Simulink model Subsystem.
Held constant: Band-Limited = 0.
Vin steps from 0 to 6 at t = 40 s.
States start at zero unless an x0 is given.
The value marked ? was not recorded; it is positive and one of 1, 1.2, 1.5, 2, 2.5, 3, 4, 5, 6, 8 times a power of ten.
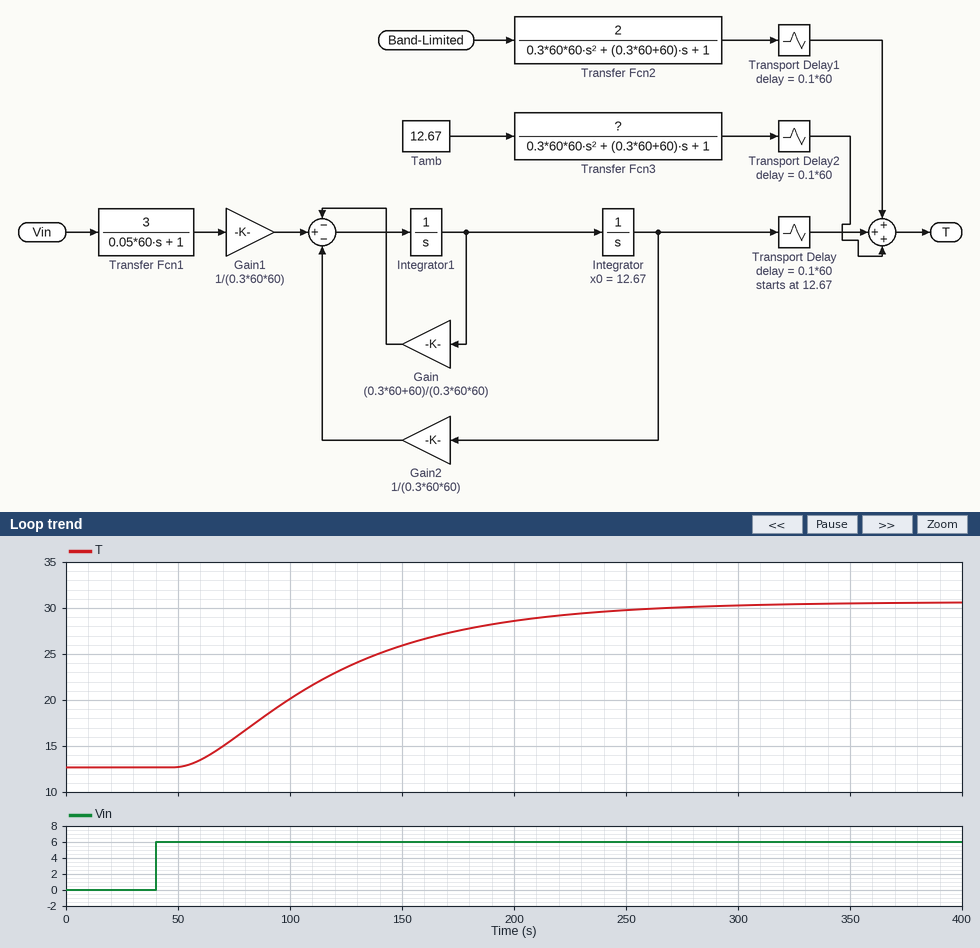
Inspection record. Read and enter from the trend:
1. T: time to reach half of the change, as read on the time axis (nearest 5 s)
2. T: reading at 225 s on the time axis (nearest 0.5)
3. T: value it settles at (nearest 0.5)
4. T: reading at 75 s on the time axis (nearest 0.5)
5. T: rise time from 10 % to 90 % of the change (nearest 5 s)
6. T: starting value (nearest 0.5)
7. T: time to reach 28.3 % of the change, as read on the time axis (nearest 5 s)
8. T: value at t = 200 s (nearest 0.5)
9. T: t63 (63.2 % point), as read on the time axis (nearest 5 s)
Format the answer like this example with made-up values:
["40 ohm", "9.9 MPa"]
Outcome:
["110 s", "29.5", "30.5", "16.0", "140 s", "12.5", "85 s", "28.5", "130 s"]
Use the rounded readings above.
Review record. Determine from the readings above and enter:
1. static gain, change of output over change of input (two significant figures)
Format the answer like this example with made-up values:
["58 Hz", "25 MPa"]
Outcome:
["3.0"]
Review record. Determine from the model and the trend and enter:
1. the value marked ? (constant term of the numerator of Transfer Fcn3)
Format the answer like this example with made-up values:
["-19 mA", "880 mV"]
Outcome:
["1"]
